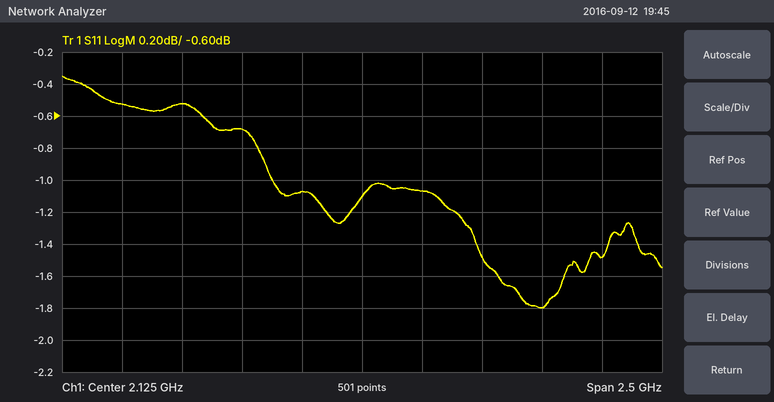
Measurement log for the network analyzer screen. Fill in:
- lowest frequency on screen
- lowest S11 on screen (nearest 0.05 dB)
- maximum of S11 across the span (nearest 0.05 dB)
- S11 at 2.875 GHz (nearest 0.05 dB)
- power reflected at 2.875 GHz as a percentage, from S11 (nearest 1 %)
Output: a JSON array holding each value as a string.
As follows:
["875 MHz", "-1.80 dB", "-0.35 dB", "-1.80 dB", "66 %"]
